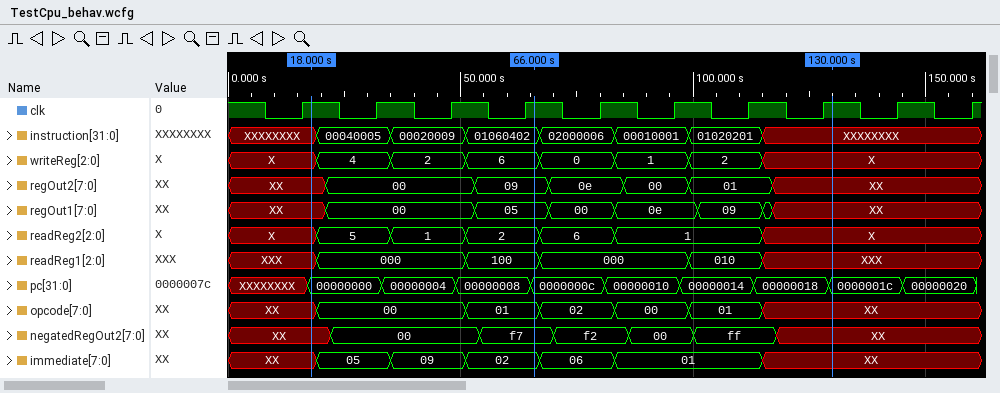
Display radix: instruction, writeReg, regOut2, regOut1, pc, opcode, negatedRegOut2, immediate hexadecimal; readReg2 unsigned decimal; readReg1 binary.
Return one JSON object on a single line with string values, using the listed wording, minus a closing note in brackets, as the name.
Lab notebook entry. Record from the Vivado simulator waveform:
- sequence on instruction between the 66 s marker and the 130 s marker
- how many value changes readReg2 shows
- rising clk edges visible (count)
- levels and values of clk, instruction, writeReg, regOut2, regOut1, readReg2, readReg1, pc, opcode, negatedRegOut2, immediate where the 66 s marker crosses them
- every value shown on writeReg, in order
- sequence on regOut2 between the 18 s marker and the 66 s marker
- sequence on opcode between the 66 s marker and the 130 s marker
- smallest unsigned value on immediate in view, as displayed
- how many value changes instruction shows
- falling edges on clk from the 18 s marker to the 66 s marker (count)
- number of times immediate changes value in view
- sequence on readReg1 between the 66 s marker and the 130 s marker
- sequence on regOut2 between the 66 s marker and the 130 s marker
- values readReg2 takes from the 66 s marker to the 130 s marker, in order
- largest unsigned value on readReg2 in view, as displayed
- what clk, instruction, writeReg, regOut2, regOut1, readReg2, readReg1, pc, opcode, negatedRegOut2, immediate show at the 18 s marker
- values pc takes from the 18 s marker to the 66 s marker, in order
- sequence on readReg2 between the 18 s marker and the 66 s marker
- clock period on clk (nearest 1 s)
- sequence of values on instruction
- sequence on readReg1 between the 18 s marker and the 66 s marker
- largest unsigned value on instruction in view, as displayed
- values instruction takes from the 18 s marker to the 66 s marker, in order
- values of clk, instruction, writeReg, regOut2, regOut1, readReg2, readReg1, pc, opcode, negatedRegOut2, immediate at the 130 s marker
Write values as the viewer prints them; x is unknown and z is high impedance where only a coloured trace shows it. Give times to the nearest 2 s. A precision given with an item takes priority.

{"sequence on instruction between the 66 s marker and the 130 s marker": "01060402, 02000006, 00010001, 01020201, XXXXXXXX", "how many value changes readReg2 shows": "6", "rising clk edges visible": "10", "levels and values of clk, instruction, writeReg, regOut2, regOut1, readReg2, readReg1, pc, opcode, negatedRegOut2, immediate where the 66 s marker crosses them": "clk=1, instruction=01060402, writeReg=6, regOut2=09, regOut1=05, readReg2=2, readReg1=100, pc=0000000c, opcode=01, negatedRegOut2=f7, immediate=02", "every value shown on writeReg, in order": "X, 4, 2, 6, 0, 1, 2, X", "sequence on regOut2 between the 18 s marker and the 66 s marker": "XX, 00, 09", "sequence on opcode between the 66 s marker and the 130 s marker": "01, 02, 00, 01, XX", "smallest unsigned value on immediate in view, as displayed": "01", "how many value changes instruction shows": "7", "falling edges on clk from the 18 s marker to the 66 s marker": "3", "number of times immediate changes value in view": "6", "sequence on readReg1 between the 66 s marker and the 130 s marker": "100, 000, 010, XXX", "sequence on regOut2 between the 66 s marker and the 130 s marker": "09, 0e, 00, 01, XX", "values readReg2 takes from the 66 s marker to the 130 s marker, in order": "2, 6, 1, X", "largest unsigned value on readReg2 in view, as displayed": "6", "what clk, instruction, writeReg, regOut2, regOut1, readReg2, readReg1, pc, opcode, negatedRegOut2, immediate show at the 18 s marker": "clk=1, instruction=XXXXXXXX, writeReg=X, regOut2=XX, regOut1=XX, readReg2=X, readReg1=XXX, pc=00000000, opcode=XX, negatedRegOut2=XX, immediate=XX", "values pc takes from the 18 s marker to the 66 s marker, in order": "00000000, 00000004, 00000008, 0000000c", "sequence on readReg2 between the 18 s marker and the 66 s marker": "X, 5, 1, 2", "clock period on clk": "16 s", "sequence of values on instruction": "XXXXXXXX, 00040005, 00020009, 01060402, 02000006, 00010001, 01020201, XXXXXXXX", "sequence on readReg1 between the 18 s marker and the 66 s marker": "XXX, 000, 100", "largest unsigned value on instruction in view, as displayed": "02000006", "values instruction takes from the 18 s marker to the 66 s marker, in order": "XXXXXXXX, 00040005, 00020009, 01060402", "values of clk, instruction, writeReg, regOut2, regOut1, readReg2, readReg1, pc, opcode, negatedRegOut2, immediate at the 130 s marker": "clk=1, instruction=XXXXXXXX, writeReg=X, regOut2=XX, regOut1=XX, readReg2=X, readReg1=XXX, pc=0000001c, opcode=XX, negatedRegOut2=XX, immediate=XX"}
